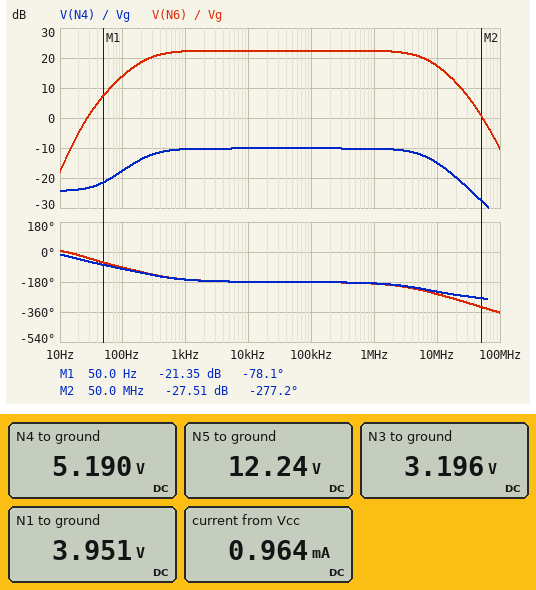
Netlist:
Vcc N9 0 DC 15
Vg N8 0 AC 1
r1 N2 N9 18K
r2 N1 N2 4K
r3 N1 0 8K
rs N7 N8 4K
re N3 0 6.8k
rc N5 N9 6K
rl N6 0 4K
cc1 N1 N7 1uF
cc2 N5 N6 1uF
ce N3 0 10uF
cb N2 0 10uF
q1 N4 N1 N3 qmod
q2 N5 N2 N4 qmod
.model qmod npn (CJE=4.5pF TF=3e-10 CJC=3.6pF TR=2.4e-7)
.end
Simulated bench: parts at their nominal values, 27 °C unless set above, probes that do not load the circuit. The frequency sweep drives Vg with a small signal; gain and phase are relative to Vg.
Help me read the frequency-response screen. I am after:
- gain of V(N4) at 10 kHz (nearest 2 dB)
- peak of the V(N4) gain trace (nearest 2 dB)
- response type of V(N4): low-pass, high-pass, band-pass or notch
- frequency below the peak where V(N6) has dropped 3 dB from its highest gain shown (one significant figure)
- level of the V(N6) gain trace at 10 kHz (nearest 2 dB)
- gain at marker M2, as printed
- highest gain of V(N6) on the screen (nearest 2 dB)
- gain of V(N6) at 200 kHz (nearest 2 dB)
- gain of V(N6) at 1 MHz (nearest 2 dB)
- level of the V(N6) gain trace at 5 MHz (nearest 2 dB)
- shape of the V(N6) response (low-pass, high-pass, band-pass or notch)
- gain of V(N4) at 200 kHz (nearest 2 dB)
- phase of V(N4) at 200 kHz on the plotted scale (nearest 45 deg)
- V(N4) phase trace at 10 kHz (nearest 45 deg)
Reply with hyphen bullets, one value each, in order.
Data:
- -10 dB
- -10 dB
- band-pass
- 200 Hz
- 22 dB
- -27.51 dB
- 22 dB
- 22 dB
- 22 dB
- 20 dB
- band-pass
- -10 dB
- -180 deg
- -180 deg
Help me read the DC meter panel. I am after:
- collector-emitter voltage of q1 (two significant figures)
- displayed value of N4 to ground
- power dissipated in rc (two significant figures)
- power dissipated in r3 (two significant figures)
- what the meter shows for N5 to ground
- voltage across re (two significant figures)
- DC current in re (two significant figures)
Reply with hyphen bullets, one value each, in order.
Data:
- 2.0 V
- 5.190 V
- 1.3 mW
- 2.0 mW
- 12.24 V
- 3.2 V
- 470 µA
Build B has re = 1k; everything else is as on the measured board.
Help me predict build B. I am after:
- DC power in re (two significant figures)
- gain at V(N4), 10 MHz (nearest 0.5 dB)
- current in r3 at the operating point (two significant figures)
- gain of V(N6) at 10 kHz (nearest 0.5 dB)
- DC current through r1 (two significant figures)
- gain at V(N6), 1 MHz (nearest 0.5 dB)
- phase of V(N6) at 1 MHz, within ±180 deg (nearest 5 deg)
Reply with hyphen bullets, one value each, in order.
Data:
- 4.4 mW
- -21.5 dB
- 360 µA
- 5.5 dB
- 590 µA
- 0.5 dB
- 115 deg
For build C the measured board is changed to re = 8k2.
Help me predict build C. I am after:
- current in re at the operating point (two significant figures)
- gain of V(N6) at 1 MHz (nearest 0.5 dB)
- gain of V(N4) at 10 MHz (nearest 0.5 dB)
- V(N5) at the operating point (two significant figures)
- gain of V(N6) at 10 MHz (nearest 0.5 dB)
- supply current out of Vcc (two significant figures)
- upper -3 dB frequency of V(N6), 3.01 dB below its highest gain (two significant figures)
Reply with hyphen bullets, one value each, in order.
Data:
- 390 µA
- 21.0 dB
- -14.5 dB
- 13 V
- 16.0 dB
- 890 µA
- 6.9 MHz
